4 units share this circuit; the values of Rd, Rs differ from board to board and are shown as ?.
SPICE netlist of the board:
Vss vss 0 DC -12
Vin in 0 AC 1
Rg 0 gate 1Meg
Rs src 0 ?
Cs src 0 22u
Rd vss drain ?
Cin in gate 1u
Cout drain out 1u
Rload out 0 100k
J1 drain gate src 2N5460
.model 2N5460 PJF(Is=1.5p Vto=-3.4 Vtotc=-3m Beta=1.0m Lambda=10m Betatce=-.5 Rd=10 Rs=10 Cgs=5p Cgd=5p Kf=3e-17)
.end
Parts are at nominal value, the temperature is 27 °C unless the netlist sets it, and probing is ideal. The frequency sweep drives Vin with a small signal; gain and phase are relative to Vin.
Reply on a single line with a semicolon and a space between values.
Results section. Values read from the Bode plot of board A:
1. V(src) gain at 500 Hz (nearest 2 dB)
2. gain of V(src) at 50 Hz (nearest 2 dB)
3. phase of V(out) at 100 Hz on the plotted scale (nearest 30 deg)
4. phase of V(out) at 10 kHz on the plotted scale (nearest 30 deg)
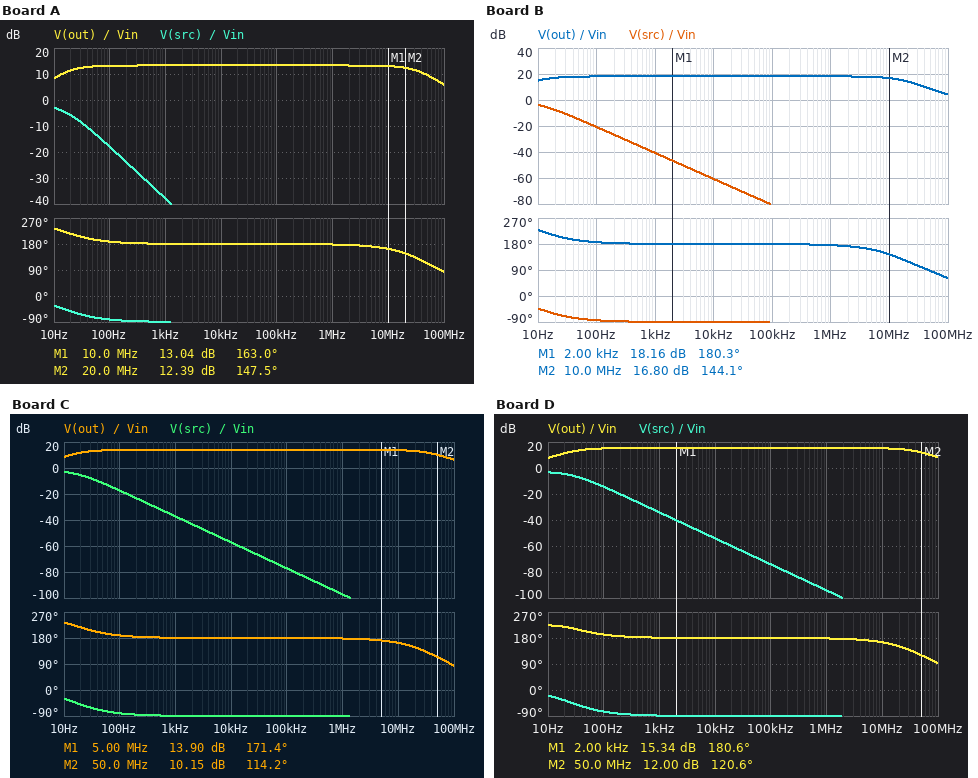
-32 dB; -12 dB; 180 deg; 180 deg
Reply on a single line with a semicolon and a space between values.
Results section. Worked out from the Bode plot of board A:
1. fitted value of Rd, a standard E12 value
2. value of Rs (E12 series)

2.7 kΩ; 3.3 kΩ
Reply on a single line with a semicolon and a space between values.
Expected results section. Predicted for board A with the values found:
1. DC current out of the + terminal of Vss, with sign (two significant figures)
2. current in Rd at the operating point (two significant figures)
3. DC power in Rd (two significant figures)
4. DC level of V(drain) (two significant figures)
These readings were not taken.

-770 µA; 770 µA; 1.6 mW; -9.9 V
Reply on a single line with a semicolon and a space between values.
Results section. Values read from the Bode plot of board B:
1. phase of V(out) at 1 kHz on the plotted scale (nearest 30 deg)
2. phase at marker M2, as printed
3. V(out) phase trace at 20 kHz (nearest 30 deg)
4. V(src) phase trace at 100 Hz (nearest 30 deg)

180 deg; 144.1 deg; 180 deg; -90 deg
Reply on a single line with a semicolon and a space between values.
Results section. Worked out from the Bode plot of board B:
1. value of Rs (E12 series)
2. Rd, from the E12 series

6.8 kΩ; 6.8 kΩ
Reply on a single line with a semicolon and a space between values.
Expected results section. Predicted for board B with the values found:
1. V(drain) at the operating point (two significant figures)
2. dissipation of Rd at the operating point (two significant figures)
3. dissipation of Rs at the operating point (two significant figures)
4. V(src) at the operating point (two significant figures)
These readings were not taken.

-9.2 V; 1.1 mW; 1.1 mW; -2.8 V
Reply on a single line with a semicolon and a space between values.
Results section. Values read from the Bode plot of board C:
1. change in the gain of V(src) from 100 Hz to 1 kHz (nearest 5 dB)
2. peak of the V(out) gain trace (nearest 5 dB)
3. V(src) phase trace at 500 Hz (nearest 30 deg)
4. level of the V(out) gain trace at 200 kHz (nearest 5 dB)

-20 dB; 15 dB; -90 deg; 15 dB
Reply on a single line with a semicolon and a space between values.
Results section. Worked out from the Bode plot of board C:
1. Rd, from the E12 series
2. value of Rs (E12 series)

2.7 kΩ; 2.7 kΩ
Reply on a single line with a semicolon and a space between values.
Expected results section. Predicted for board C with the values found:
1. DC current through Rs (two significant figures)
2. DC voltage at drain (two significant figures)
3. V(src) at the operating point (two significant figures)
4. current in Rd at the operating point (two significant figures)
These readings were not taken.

910 µA; -9.5 V; -2.5 V; 910 µA
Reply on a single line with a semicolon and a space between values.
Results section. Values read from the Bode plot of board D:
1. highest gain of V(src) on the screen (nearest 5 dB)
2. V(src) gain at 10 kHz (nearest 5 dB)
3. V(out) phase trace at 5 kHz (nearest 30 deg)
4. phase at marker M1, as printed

-5 dB; -55 dB; 180 deg; 180.6 deg
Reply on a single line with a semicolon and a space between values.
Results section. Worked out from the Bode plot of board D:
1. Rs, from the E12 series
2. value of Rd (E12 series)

1 kΩ; 2.2 kΩ
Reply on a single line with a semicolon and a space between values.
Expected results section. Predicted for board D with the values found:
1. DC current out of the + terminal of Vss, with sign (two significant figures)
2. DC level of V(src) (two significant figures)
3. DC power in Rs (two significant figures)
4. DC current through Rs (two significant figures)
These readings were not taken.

-2.0 mA; -2.0 V; 4.0 mW; 2.0 mA
